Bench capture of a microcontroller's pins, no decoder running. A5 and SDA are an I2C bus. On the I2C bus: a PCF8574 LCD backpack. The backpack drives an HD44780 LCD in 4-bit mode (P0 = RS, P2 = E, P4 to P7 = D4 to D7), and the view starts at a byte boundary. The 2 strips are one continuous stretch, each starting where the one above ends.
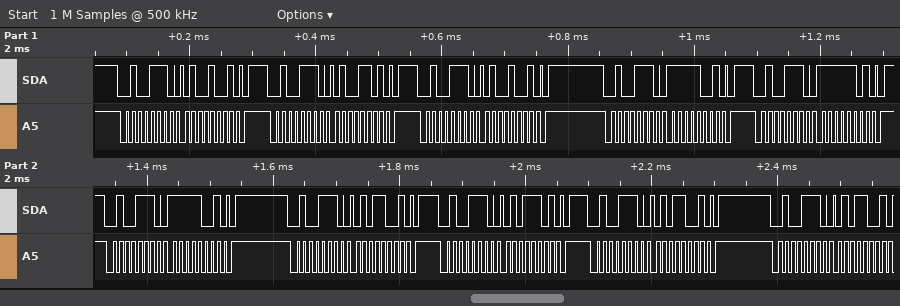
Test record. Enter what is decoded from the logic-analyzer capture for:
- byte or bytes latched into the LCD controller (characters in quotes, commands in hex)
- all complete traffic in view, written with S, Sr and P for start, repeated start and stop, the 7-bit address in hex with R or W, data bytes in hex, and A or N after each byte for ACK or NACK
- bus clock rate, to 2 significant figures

'O'
S 27W A 49 A P S 27W A 4D A P S 27W A 49 A P S 27W A F9 A P S 27W A FD A P S 27W A F9 A P S 27W A 59 A P S 27W A 5D A P S 27W A 59 A P S 27W A 59 A
100 kHz
